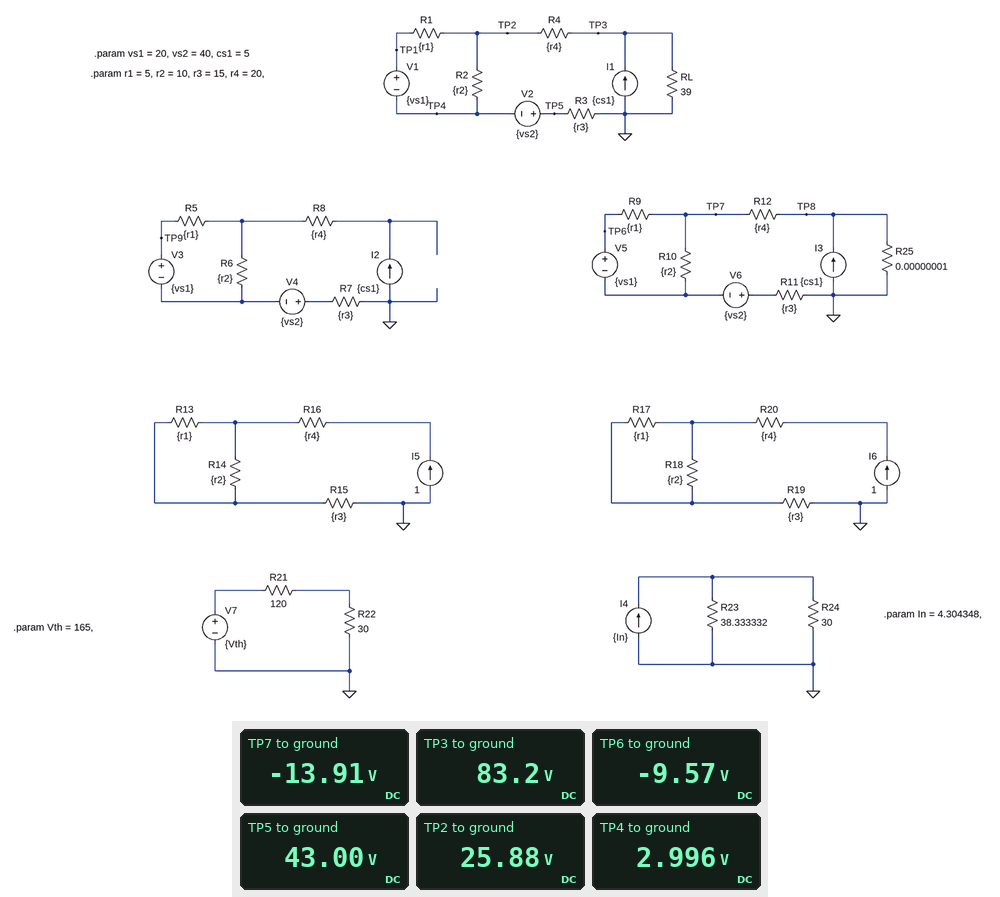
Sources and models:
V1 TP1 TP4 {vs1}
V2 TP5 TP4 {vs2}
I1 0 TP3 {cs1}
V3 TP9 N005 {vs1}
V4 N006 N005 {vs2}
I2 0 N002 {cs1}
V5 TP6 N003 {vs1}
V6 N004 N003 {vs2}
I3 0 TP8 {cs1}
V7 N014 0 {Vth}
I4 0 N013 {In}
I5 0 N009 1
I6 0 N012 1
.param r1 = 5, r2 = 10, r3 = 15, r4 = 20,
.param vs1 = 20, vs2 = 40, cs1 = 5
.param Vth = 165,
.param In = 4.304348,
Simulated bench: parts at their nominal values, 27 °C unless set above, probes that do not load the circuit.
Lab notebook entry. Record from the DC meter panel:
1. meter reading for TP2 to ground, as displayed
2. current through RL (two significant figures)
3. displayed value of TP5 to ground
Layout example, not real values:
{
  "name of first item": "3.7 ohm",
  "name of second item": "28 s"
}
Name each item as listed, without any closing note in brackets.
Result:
{
  "meter reading for TP2 to ground, as displayed": "25.88 V",
  "current through RL": "2.1 A",
  "displayed value of TP5 to ground": "43.00 V"
}
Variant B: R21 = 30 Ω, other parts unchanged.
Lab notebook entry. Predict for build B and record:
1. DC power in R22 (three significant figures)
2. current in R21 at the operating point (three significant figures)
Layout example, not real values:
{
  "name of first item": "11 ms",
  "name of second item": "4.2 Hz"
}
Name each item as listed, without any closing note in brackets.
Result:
{
  "DC power in R22": "227 W",
  "current in R21 at the operating point": "2.75 A"
}
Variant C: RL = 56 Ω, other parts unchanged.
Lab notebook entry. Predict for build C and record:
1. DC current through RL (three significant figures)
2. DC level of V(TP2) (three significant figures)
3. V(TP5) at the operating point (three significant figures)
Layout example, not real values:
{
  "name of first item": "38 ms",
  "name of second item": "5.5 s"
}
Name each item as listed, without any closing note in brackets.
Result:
{
  "DC current through RL": "1.75 A",
  "DC level of V(TP2)": "32.9 V",
  "V(TP5) at the operating point": "48.8 V"
}
